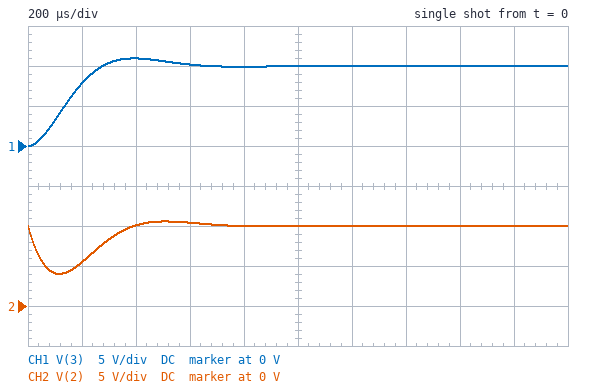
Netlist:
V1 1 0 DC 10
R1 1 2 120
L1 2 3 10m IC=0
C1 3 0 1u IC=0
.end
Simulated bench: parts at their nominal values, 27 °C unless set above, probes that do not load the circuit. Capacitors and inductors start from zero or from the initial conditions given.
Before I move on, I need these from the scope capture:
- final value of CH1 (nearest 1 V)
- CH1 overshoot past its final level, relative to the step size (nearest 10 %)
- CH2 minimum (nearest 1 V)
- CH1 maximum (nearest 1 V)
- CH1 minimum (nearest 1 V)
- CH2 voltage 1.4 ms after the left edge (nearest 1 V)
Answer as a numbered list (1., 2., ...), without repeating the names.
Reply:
1. 10 V
2. 10 %
3. 4 V
4. 11 V
5. 0 V
6. 10 V
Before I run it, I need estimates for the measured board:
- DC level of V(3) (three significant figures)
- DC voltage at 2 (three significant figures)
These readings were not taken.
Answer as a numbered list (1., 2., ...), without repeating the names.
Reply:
1. 10.0 V
2. 10.0 V
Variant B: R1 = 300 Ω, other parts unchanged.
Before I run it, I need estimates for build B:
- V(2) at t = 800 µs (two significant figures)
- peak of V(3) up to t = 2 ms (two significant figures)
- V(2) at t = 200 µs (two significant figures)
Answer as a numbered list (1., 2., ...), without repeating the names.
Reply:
1. 9.4 V
2. 10 V
3. 3.8 V
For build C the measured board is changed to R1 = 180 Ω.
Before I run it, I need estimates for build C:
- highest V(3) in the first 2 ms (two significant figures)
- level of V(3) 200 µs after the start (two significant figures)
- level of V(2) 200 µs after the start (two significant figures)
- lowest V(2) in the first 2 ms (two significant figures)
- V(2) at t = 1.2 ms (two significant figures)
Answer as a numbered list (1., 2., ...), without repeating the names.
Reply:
1. 10 V
2. 6.3 V
3. 4.8 V
4. 2.9 V
5. 10 V
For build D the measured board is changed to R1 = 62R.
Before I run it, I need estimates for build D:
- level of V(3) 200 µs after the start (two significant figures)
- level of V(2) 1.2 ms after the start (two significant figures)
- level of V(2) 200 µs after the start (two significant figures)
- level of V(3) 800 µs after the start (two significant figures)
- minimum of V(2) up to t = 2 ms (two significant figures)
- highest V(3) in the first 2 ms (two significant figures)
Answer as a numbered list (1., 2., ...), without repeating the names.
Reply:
1. 10 V
2. 10 V
3. 6.7 V
4. 9.5 V
5. 5.9 V
6. 14 V
